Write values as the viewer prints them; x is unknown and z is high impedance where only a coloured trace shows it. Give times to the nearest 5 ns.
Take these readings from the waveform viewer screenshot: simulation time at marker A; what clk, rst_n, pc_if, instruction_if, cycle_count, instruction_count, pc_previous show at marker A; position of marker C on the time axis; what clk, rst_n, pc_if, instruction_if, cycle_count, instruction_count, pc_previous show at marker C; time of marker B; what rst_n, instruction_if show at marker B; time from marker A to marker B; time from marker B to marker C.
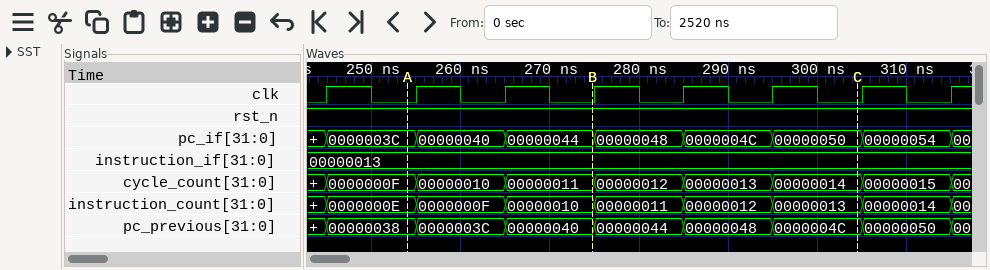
255 ns
clk=0, rst_n=1, pc_if=0000003C, instruction_if=00000013, cycle_count=0000000F, instruction_count=0000000E, pc_previous=00000038
305 ns
clk=0, rst_n=1, pc_if=00000050, instruction_if=00000013, cycle_count=00000014, instruction_count=00000013, pc_previous=0000004C
275 ns
rst_n=1, instruction_if=00000013
20 ns
30 ns
